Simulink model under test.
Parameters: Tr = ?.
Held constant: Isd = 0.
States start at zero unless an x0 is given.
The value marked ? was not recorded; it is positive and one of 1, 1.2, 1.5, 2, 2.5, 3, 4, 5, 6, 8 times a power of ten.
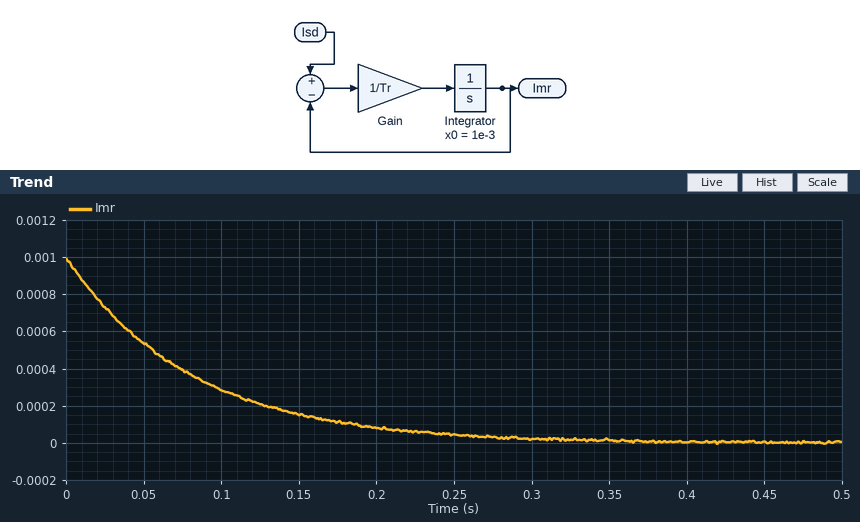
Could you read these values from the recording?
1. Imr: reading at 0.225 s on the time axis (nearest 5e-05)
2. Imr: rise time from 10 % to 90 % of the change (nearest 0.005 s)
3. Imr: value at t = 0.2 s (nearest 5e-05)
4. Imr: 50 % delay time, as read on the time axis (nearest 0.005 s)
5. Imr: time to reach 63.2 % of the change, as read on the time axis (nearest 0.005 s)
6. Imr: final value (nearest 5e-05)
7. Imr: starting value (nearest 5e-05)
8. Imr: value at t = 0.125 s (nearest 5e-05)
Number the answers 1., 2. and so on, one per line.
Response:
1. 0.00005
2. 0.175 s
3. 0.00010
4. 0.055 s
5. 0.080 s
6. 0.00000
7. 0.00100
8. 0.00020
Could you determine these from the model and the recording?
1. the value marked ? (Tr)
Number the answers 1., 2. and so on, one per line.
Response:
1. 0.08
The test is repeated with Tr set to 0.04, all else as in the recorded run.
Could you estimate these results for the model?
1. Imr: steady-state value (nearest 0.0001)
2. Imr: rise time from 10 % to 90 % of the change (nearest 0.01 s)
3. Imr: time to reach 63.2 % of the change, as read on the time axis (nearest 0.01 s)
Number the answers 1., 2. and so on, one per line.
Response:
1. 0.0000
2. 0.09 s
3. 0.04 s
